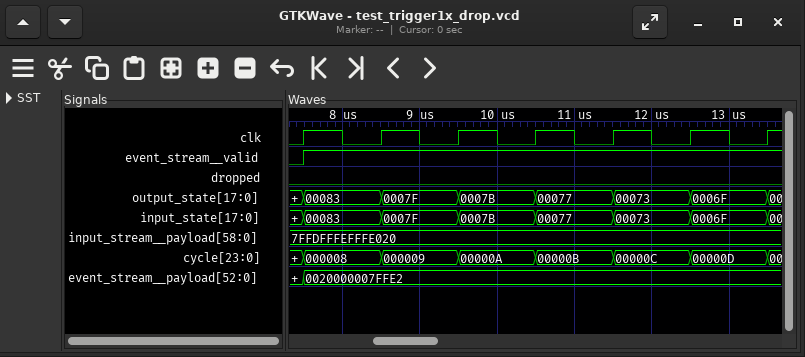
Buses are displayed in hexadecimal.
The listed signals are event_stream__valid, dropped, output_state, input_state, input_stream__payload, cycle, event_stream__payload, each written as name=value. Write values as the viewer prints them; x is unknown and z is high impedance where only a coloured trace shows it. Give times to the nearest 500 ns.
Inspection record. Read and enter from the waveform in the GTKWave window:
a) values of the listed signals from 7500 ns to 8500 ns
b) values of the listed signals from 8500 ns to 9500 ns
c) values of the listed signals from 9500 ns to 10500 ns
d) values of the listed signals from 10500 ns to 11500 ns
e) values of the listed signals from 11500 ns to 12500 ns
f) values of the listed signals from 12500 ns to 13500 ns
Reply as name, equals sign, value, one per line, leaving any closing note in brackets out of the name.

values of the listed signals from 7500 ns to 8500 ns = event_stream__valid=1, dropped=0, output_state=00083, input_state=00083, input_stream__payload=7FFDFFFEFFFE020, cycle=000008, event_stream__payload=0020000007FFE2
values of the listed signals from 8500 ns to 9500 ns = event_stream__valid=1, dropped=0, output_state=0007F, input_state=0007F, input_stream__payload=7FFDFFFEFFFE020, cycle=000009, event_stream__payload=0020000007FFE2
values of the listed signals from 9500 ns to 10500 ns = event_stream__valid=1, dropped=0, output_state=0007B, input_state=0007B, input_stream__payload=7FFDFFFEFFFE020, cycle=00000A, event_stream__payload=0020000007FFE2
values of the listed signals from 10500 ns to 11500 ns = event_stream__valid=1, dropped=0, output_state=00077, input_state=00077, input_stream__payload=7FFDFFFEFFFE020, cycle=00000B, event_stream__payload=0020000007FFE2
values of the listed signals from 11500 ns to 12500 ns = event_stream__valid=1, dropped=0, output_state=00073, input_state=00073, input_stream__payload=7FFDFFFEFFFE020, cycle=00000C, event_stream__payload=0020000007FFE2
values of the listed signals from 12500 ns to 13500 ns = event_stream__valid=1, dropped=0, output_state=0006F, input_state=0006F, input_stream__payload=7FFDFFFEFFFE020, cycle=00000D, event_stream__payload=0020000007FFE2
